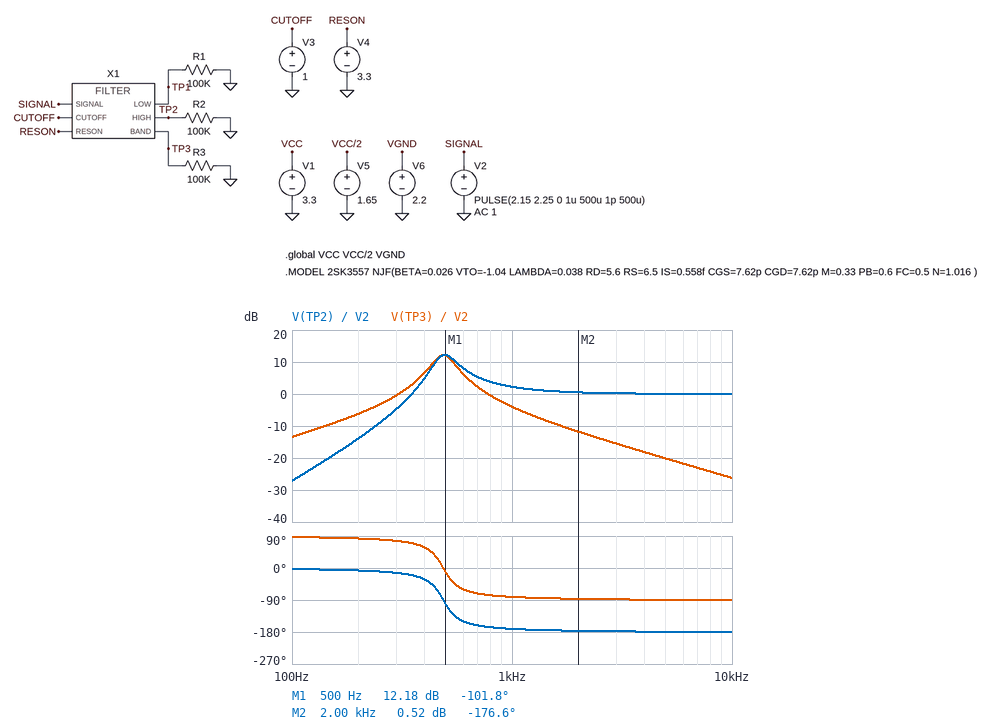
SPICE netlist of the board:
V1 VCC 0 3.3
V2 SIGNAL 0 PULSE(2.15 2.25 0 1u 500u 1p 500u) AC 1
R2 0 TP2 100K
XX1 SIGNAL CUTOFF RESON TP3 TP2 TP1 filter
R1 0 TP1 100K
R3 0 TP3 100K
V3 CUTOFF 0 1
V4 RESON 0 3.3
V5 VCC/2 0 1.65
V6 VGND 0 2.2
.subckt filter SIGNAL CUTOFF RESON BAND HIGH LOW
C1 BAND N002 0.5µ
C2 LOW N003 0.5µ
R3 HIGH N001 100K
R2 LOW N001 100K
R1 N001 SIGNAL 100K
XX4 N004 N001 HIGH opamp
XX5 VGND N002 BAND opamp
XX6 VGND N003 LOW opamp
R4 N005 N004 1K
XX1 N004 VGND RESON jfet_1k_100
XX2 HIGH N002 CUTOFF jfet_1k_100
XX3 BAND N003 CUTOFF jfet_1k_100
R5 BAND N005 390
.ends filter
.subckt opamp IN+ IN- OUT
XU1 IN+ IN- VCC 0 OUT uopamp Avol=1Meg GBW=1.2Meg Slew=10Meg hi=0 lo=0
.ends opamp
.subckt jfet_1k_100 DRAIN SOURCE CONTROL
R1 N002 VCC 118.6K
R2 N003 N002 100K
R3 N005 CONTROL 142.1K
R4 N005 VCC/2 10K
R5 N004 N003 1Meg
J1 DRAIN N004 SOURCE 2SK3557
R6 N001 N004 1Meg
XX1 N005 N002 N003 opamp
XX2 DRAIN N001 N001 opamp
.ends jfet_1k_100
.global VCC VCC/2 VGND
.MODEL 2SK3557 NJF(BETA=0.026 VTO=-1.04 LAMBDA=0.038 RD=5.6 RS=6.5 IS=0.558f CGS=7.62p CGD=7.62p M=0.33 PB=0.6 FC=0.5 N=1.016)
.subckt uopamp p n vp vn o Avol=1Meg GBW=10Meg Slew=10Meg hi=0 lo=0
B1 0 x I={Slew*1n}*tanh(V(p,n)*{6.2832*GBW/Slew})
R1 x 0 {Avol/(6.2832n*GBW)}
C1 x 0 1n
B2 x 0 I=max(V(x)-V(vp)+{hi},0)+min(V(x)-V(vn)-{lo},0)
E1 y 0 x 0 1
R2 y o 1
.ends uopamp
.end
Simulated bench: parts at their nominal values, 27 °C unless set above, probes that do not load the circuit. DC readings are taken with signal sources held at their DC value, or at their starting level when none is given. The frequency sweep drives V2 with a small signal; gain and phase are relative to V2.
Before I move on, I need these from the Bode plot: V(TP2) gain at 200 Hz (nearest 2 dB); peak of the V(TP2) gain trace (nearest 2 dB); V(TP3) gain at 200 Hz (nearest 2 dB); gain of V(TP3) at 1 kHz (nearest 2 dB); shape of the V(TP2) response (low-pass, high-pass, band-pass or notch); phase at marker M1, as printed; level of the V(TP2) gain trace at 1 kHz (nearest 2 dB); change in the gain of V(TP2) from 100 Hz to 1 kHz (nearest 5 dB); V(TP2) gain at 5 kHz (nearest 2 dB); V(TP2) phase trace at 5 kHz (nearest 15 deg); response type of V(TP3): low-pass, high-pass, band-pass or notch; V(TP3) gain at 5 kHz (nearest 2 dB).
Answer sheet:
-14 dB
12 dB
-6 dB
-4 dB
high-pass
-101.8 deg
2 dB
30 dB
0 dB
-180 deg
band-pass
-20 dB
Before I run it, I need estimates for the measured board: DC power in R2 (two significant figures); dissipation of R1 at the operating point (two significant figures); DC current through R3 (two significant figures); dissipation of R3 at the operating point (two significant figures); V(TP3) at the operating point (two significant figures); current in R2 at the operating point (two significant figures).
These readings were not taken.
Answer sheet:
48 µW
51 µW
22 µA
48 µW
2.2 V
22 µA
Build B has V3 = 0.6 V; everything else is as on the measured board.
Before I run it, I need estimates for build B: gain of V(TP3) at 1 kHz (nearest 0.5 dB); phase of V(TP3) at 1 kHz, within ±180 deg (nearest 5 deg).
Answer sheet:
-20.5 dB
-90 deg
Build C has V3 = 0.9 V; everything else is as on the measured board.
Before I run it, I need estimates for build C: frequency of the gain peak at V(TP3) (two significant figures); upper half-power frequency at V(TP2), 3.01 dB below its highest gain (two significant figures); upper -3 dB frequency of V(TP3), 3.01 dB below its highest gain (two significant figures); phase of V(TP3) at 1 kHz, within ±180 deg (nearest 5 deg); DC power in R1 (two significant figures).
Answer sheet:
390 Hz
460 Hz
440 Hz
-85 deg
51 µW
